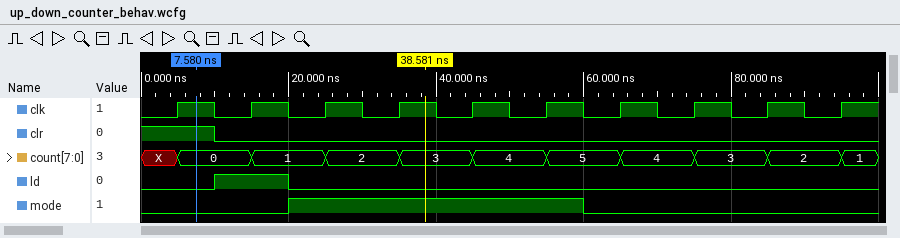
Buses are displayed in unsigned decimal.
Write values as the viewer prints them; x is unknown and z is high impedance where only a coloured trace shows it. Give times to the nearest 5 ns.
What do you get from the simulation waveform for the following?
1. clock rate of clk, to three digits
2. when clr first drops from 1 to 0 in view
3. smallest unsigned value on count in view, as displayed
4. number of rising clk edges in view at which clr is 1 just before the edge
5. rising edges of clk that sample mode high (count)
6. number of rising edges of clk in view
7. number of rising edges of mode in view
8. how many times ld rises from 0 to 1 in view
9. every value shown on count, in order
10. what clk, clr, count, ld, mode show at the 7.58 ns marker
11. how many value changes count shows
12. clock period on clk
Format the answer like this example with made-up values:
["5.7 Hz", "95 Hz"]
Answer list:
["100 MHz", "10 ns", "0", "1", "4", "10", "1", "1", "X, 0, 1, 2, 3, 4, 5, 4, 3, 2, 1", "clk=1, clr=1, count=0, ld=0, mode=0", "10", "10 ns"]
